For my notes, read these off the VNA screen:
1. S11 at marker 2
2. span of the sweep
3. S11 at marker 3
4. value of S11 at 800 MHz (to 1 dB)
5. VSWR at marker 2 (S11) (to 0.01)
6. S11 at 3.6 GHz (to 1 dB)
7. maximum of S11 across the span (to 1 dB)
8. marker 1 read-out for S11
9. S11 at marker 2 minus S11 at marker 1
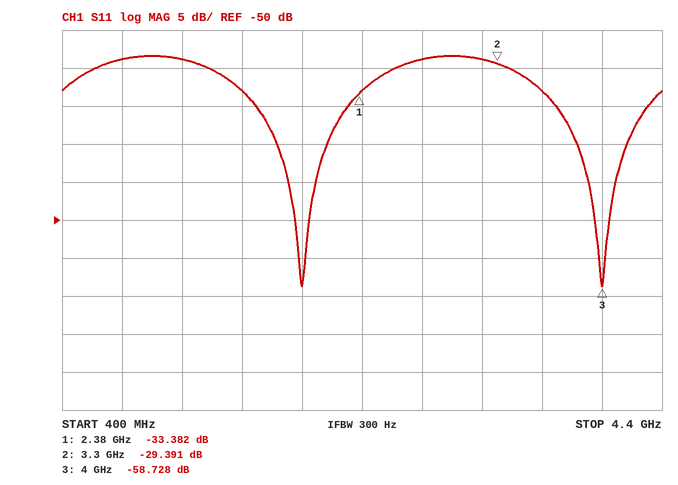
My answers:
-29.391 dB
4 GHz
-58.728 dB
-29 dB
1.07
-33 dB
-28 dB
-33.382 dB
3.991 dB
